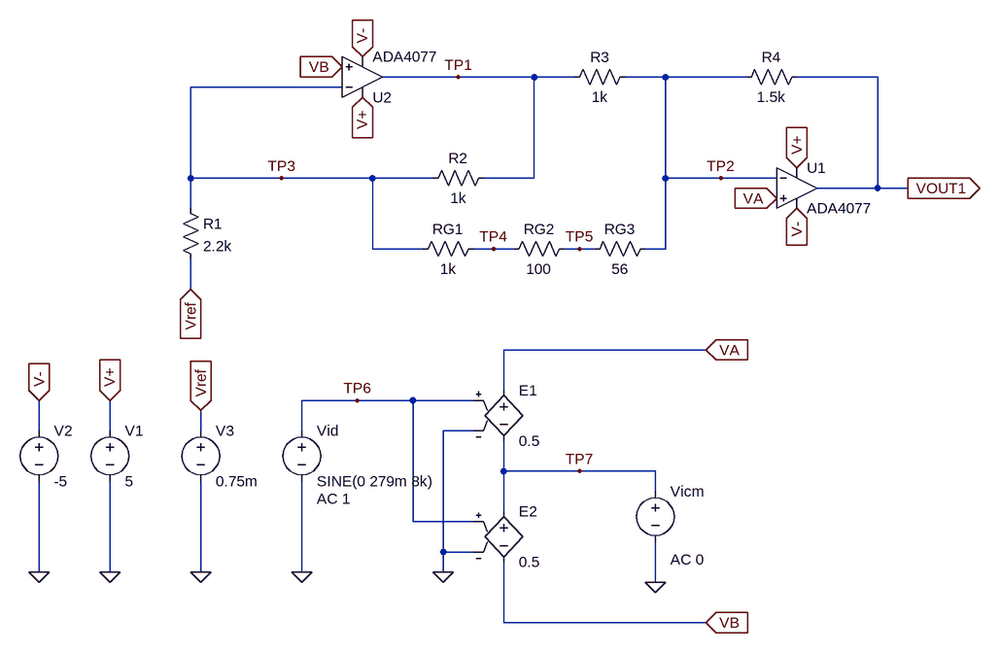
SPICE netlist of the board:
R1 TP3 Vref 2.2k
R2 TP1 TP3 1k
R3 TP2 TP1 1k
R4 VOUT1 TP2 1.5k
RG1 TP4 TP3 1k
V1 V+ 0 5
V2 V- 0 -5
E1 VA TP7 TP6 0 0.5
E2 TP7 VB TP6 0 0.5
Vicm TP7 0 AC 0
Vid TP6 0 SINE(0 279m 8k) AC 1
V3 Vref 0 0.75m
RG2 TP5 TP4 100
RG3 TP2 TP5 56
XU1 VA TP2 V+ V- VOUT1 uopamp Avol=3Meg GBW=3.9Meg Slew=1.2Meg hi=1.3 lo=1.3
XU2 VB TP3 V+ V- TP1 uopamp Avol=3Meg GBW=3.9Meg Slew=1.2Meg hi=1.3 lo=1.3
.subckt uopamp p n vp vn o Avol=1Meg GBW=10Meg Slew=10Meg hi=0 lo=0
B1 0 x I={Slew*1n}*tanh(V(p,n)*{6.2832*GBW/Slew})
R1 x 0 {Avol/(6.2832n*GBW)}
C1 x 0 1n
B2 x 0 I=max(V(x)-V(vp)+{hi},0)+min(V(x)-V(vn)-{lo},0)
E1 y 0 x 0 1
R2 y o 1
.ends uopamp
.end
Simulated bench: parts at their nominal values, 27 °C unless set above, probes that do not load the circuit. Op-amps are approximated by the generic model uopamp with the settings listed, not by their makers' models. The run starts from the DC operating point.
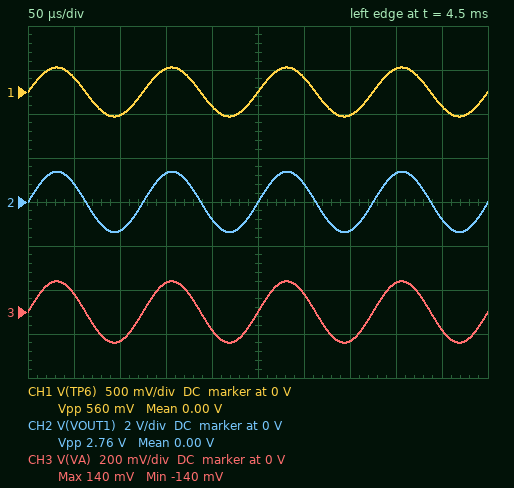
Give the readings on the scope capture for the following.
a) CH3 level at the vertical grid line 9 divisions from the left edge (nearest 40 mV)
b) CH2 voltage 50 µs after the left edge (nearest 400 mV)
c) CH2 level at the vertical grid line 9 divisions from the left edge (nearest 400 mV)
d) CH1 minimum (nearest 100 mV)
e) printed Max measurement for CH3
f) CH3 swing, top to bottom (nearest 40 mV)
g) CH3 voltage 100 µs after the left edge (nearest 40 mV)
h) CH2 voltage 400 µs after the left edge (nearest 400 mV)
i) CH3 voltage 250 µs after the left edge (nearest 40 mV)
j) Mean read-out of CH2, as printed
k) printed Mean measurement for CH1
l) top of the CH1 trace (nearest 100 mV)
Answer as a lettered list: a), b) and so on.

a) -80 mV
b) 800 mV
c) -800 mV
d) -300 mV
e) 140 mV
f) 280 mV
g) -120 mV
h) 1.2 V
i) 0 V
j) 0.00 V
k) 0.00 V
l) 300 mV
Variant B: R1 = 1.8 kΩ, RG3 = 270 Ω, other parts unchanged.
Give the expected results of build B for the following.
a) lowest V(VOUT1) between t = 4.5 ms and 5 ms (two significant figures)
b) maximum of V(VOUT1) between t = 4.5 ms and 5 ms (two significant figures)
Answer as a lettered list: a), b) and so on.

a) -1.3 V
b) 1.3 V
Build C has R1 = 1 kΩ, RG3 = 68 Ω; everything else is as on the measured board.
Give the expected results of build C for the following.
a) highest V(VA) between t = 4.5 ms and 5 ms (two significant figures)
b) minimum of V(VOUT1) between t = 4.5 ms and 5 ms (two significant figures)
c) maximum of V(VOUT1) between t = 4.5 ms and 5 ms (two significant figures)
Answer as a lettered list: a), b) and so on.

a) 140 mV
b) -1.5 V
c) 1.5 V
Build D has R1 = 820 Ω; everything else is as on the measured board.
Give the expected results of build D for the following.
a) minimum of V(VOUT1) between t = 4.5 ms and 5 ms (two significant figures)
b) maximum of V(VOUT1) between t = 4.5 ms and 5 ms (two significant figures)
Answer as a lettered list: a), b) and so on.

a) -1.5 V
b) 1.5 V
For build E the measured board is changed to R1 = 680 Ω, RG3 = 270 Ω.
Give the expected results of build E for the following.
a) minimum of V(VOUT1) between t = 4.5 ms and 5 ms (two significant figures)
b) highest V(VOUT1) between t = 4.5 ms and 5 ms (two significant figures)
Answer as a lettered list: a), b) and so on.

a) -1.5 V
b) 1.5 V
